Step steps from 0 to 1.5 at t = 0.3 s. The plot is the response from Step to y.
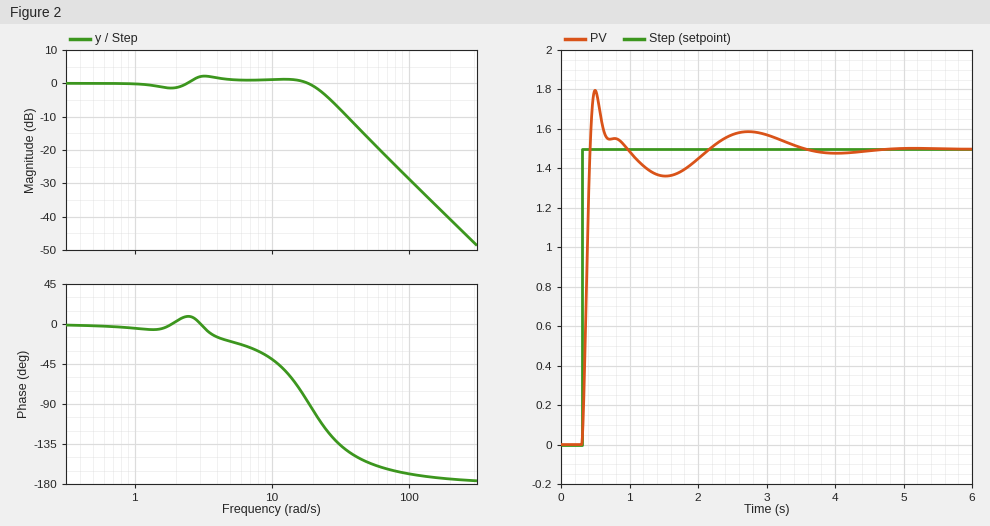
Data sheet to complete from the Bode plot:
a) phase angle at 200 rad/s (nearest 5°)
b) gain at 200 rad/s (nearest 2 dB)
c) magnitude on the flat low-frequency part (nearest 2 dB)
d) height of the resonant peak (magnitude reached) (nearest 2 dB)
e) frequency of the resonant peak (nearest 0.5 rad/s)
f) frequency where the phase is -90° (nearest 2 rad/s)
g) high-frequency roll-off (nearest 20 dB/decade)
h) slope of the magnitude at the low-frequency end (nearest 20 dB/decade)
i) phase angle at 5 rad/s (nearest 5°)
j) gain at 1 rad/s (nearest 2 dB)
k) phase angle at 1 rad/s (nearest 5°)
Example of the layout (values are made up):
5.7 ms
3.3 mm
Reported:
-175°
-40 dB
0 dB
2 dB
3.5 rad/s
18 rad/s
-40 dB/decade
0 dB/decade
-20°
0 dB
-5°
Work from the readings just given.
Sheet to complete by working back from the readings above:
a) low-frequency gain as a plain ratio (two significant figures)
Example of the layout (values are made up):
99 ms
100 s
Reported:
1.0
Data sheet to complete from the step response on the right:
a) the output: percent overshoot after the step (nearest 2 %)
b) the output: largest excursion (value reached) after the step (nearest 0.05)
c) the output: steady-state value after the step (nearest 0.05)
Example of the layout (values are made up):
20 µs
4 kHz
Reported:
20 %
1.80
1.50
